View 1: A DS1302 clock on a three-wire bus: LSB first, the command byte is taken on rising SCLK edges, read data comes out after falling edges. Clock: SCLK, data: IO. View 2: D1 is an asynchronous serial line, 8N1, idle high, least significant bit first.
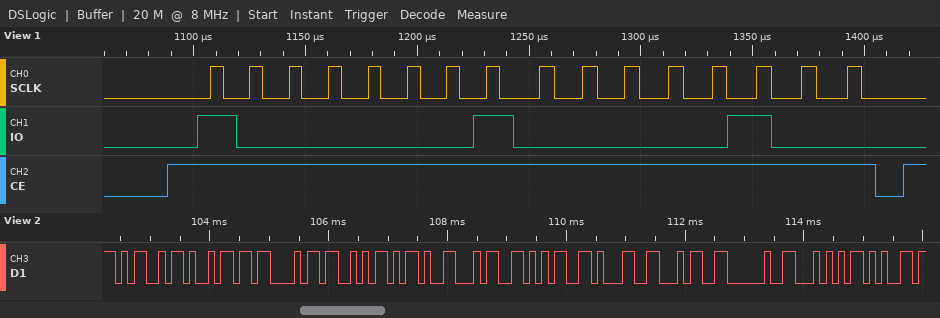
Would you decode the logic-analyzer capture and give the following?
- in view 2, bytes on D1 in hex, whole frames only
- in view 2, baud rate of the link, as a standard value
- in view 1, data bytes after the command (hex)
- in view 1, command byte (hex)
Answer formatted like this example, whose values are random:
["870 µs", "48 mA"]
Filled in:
["4D 69 43 53 2D 34 35 31 34 20 54 65", "9600 baud", "20", "0x81"]
